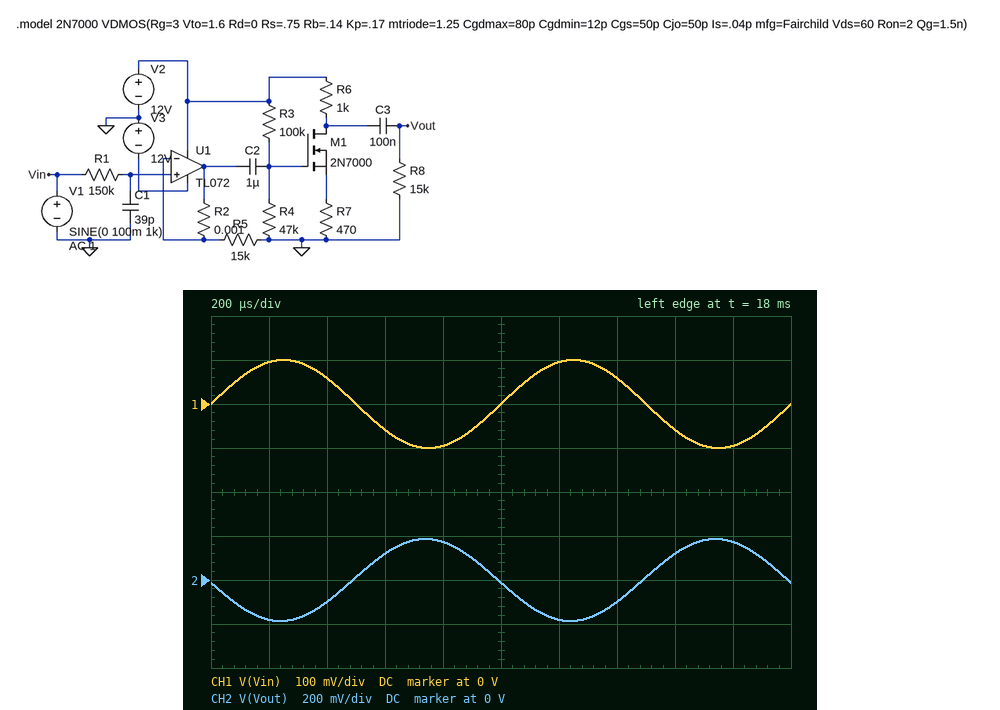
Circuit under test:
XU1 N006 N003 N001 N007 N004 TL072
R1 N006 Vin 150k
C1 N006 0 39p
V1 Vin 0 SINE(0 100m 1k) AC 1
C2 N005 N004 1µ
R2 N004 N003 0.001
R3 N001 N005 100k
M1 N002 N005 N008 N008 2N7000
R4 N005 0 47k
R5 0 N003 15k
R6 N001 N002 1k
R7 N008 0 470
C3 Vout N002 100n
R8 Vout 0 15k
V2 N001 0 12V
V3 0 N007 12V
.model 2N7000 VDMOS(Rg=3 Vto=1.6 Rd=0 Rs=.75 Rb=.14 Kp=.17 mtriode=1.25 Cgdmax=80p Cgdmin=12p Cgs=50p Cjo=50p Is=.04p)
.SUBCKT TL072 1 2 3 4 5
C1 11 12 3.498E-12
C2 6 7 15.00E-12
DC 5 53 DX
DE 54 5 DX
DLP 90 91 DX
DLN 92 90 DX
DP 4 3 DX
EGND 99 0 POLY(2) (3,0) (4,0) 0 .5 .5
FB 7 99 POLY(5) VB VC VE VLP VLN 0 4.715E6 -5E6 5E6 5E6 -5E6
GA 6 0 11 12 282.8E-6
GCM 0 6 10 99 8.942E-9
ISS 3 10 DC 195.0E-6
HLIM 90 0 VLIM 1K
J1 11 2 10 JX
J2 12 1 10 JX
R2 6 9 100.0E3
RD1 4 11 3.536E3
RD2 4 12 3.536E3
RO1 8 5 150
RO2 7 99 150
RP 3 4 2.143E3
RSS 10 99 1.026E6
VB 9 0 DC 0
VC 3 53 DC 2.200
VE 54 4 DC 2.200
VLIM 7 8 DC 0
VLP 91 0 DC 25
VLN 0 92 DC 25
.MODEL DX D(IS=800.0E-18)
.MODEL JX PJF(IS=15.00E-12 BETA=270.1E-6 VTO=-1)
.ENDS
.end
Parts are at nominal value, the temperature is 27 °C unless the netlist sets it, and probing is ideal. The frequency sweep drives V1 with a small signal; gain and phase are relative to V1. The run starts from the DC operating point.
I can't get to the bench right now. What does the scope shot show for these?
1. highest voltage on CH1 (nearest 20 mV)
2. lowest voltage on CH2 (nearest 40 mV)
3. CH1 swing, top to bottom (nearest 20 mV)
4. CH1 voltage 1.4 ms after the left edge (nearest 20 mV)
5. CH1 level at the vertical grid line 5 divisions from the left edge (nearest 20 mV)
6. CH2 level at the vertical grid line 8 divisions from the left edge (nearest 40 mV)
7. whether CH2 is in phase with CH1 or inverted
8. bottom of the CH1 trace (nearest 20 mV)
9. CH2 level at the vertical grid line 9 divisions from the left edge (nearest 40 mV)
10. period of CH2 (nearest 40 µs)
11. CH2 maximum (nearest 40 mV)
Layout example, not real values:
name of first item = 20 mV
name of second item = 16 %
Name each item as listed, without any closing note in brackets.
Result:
highest voltage on CH1 = 100 mV
lowest voltage on CH2 = -200 mV
CH1 swing, top to bottom = 200 mV
CH1 voltage 1.4 ms after the left edge = 60 mV
CH1 level at the vertical grid line 5 divisions from the left edge = 0 V
CH2 level at the vertical grid line 8 divisions from the left edge = 120 mV
whether CH2 is in phase with CH1 or inverted = inverted
bottom of the CH1 trace = -100 mV
CH2 level at the vertical grid line 9 divisions from the left edge = 160 mV
period of CH2 = 1.00 ms
CH2 maximum = 200 mV
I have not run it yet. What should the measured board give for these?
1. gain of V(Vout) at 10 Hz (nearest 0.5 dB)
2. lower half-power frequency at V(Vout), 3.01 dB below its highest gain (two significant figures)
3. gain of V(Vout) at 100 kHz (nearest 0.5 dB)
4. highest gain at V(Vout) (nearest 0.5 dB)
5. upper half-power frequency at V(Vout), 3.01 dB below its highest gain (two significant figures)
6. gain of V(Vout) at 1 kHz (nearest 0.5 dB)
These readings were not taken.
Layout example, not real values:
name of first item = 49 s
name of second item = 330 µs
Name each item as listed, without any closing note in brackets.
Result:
gain of V(Vout) at 10 Hz = -15.5 dB
lower half-power frequency at V(Vout), 3.01 dB below its highest gain = 99 Hz
gain of V(Vout) at 100 kHz = -6.0 dB
highest gain at V(Vout) = 5.5 dB
upper half-power frequency at V(Vout), 3.01 dB below its highest gain = 27 kHz
gain of V(Vout) at 1 kHz = 5.5 dB
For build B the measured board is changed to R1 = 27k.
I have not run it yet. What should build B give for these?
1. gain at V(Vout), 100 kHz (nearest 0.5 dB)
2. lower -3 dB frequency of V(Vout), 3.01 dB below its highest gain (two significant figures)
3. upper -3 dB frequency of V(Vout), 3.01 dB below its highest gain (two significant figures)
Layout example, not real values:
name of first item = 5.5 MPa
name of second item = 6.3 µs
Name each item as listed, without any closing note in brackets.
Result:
gain at V(Vout), 100 kHz = 4.0 dB
lower -3 dB frequency of V(Vout), 3.01 dB below its highest gain = 100 Hz
upper -3 dB frequency of V(Vout), 3.01 dB below its highest gain = 150 kHz
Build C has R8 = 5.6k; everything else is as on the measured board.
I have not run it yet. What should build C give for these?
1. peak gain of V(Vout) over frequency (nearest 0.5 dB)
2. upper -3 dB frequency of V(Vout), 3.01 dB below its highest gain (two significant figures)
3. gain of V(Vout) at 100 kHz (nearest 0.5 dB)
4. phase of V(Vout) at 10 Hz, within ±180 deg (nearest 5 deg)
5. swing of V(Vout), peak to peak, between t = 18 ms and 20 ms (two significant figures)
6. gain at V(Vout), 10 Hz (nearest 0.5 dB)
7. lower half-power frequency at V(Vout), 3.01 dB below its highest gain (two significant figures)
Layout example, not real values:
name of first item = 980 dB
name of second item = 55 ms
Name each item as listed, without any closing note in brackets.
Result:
peak gain of V(Vout) over frequency = 4.5 dB
upper -3 dB frequency of V(Vout), 3.01 dB below its highest gain = 28 kHz
gain of V(Vout) at 100 kHz = -7.0 dB
phase of V(Vout) at 10 Hz, within ±180 deg = -65 deg
swing of V(Vout), peak to peak, between t = 18 ms and 20 ms = 330 mV
gain at V(Vout), 10 Hz = -24.0 dB
lower half-power frequency at V(Vout), 3.01 dB below its highest gain = 240 Hz
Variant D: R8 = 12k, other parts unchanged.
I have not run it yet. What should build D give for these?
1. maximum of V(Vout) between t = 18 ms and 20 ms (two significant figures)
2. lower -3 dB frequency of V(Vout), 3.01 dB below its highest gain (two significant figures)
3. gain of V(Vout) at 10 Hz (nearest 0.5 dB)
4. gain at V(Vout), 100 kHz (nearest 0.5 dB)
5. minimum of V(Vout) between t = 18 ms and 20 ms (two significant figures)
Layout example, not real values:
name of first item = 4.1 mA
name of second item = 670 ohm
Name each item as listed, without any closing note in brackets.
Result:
maximum of V(Vout) between t = 18 ms and 20 ms = 180 mV
lower -3 dB frequency of V(Vout), 3.01 dB below its highest gain = 120 Hz
gain of V(Vout) at 10 Hz = -17.5 dB
gain at V(Vout), 100 kHz = -6.5 dB
minimum of V(Vout) between t = 18 ms and 20 ms = -180 mV
